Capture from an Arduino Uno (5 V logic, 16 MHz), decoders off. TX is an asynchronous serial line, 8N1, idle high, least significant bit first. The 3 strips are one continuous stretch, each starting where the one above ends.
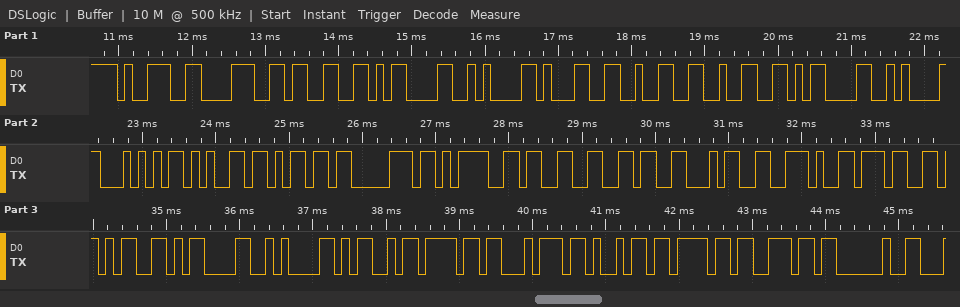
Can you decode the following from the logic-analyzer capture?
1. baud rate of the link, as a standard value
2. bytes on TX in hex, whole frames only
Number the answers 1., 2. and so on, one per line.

1. 9600 baud
2. 39 38 33 0D 0A 31 32 32 0D 0A 54 65 6D 70 3D 33 36 34 2E 37 35 0D 0A 4D 6F 74 69 6F 6E 20
